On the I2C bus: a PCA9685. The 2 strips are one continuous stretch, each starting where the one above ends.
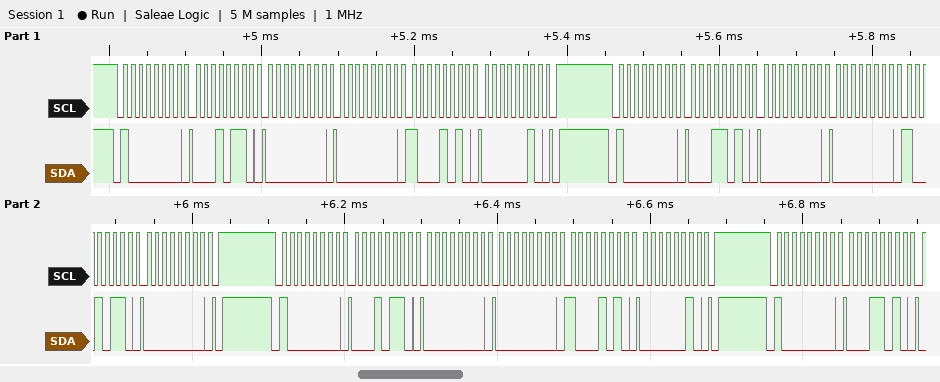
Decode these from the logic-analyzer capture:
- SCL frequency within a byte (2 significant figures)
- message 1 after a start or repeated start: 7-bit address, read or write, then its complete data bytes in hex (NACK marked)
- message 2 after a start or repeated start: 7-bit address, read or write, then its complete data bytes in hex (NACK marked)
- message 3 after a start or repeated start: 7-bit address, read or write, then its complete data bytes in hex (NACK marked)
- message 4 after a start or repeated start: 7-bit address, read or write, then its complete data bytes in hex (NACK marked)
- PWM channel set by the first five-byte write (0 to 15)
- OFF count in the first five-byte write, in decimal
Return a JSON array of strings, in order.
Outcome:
["100 kHz", "0x40 write: 16 00 00 8A 02", "0x40 write: 1A 00 00 96 00", "0x40 write: 16 00 00 8A 02", "0x40 write: 1A", "4", "650"]
